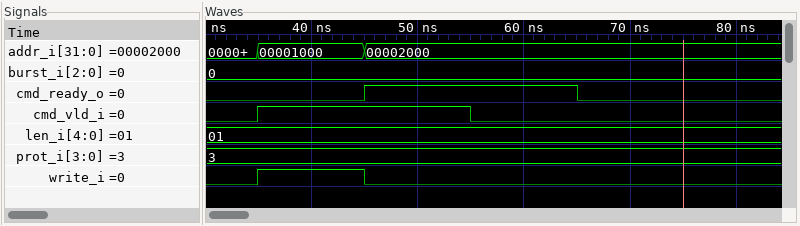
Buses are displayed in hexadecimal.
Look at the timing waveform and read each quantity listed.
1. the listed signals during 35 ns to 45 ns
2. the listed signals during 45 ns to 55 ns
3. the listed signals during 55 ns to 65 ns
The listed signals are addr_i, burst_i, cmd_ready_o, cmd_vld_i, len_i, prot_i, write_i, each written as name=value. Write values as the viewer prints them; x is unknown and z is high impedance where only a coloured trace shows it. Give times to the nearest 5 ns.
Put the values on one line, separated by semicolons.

addr_i=00001000, burst_i=0, cmd_ready_o=0, cmd_vld_i=1, len_i=01, prot_i=3, write_i=1; addr_i=00002000, burst_i=0, cmd_ready_o=1, cmd_vld_i=1, len_i=01, prot_i=3, write_i=0; addr_i=00002000, burst_i=0, cmd_ready_o=1, cmd_vld_i=0, len_i=01, prot_i=3, write_i=0
